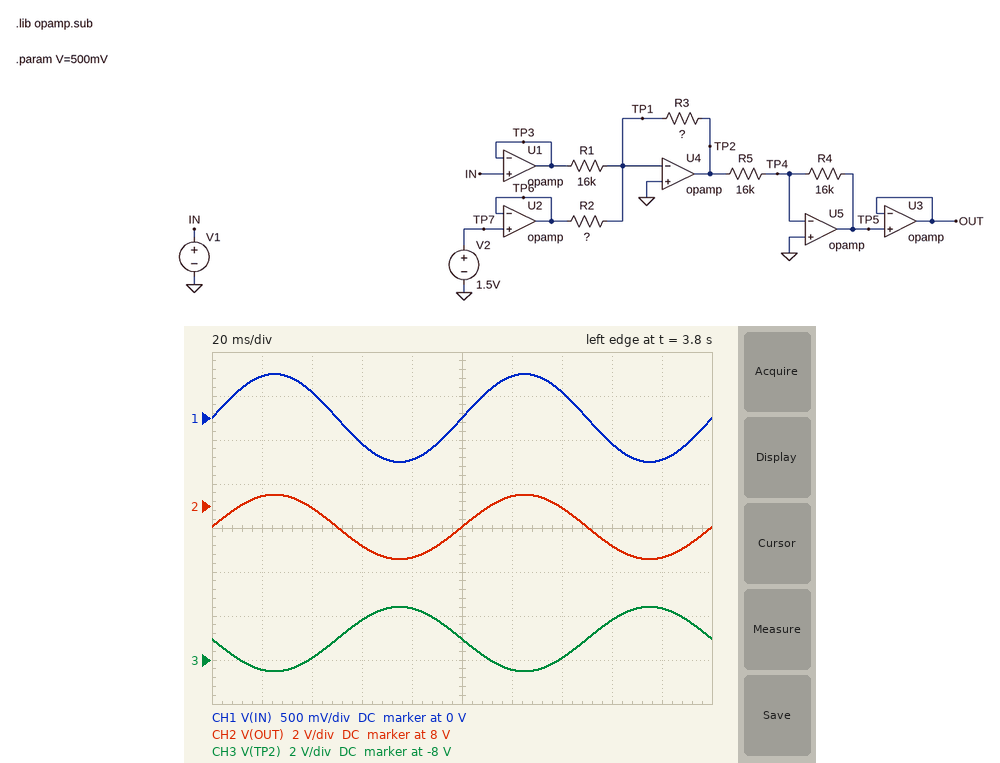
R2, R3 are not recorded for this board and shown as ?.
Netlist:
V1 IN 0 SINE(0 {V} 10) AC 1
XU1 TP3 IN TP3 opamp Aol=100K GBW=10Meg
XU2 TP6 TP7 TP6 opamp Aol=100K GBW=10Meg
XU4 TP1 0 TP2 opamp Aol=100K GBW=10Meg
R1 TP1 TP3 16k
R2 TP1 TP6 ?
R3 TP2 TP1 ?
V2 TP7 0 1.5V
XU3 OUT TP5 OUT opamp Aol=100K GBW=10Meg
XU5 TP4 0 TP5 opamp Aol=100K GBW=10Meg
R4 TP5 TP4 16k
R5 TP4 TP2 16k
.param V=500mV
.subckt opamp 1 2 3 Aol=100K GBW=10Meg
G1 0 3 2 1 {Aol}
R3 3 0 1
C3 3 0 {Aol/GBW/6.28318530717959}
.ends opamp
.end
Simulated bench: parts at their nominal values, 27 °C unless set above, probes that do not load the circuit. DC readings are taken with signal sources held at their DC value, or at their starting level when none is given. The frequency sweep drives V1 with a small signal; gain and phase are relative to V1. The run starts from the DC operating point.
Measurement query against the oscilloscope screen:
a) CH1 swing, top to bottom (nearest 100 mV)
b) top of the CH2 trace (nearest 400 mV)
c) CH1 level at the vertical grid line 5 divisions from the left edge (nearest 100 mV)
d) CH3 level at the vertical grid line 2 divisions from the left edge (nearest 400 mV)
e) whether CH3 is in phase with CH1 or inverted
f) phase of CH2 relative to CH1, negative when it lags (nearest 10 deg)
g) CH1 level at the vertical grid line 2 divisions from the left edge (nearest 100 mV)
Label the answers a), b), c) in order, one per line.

a) 1.0 V
b) 8.4 V
c) 0 V
d) -8.0 V
e) inverted
f) 0 deg
g) 300 mV
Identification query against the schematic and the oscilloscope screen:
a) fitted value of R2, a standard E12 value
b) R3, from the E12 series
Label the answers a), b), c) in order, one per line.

a) 10 kΩ
b) 47 kΩ
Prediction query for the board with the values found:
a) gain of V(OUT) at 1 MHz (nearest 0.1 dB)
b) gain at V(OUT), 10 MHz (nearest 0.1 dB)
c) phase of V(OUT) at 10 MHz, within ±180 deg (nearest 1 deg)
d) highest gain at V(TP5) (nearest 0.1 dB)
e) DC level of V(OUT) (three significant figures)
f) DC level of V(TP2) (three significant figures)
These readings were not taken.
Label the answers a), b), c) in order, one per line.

a) 6.7 dB
b) -22.4 dB
c) 123 deg
d) 9.4 dB
e) 7.05 V
f) -7.05 V
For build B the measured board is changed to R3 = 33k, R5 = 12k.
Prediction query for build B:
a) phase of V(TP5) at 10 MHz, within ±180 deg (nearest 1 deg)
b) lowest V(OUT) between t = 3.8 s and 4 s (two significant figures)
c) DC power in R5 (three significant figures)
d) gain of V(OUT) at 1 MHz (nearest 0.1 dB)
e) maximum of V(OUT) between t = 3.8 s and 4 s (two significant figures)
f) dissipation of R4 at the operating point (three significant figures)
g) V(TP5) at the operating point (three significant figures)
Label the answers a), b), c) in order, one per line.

a) 167 deg
b) 5.2 V
c) 2.04 mW
d) 7.0 dB
e) 8.0 V
f) 2.72 mW
g) 6.60 V
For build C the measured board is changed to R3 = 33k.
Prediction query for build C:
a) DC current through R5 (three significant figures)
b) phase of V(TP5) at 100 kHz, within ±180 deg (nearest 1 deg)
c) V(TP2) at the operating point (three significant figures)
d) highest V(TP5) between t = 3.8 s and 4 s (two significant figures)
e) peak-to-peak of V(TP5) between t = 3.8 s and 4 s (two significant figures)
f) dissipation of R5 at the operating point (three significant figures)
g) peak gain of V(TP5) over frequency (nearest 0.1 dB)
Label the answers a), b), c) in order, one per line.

a) 309 µA
b) -5 deg
c) -4.95 V
d) 6.0 V
e) 2.1 V
f) 1.53 mW
g) 6.3 dB
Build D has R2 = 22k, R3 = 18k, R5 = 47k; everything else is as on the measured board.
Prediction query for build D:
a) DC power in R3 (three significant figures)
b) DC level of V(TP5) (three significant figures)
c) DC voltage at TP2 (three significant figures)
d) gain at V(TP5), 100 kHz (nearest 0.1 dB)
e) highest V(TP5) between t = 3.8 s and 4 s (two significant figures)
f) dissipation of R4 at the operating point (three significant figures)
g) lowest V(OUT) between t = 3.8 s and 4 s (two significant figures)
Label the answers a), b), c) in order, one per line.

a) 83.7 µW
b) 418 mV
c) -1.23 V
d) -8.3 dB
e) 610 mV
f) 10.9 µW
g) 230 mV
